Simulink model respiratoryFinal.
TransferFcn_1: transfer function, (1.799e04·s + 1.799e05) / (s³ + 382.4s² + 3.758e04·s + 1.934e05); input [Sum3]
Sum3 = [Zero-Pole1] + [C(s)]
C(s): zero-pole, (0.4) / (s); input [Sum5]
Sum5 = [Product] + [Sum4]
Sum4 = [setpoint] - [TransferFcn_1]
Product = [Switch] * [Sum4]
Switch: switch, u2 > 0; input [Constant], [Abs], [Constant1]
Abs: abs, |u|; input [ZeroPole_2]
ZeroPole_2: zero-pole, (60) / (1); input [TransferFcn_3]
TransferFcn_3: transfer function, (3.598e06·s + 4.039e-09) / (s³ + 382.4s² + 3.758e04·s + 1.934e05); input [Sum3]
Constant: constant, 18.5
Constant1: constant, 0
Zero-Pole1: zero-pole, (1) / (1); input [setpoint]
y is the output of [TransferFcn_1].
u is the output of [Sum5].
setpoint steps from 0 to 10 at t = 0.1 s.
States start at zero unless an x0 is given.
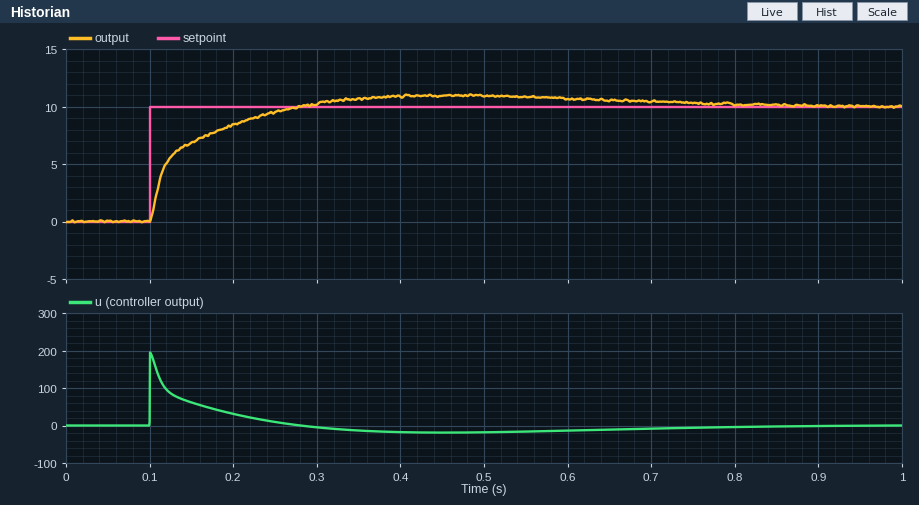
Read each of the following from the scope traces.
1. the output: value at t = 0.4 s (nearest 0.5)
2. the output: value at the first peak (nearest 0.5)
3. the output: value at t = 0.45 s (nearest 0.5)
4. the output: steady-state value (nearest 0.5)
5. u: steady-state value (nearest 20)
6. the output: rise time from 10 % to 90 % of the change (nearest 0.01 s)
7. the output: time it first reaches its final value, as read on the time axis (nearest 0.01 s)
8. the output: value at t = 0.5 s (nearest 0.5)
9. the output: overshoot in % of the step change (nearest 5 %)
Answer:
11.0
11.0
11.0
10.0
0
0.12 s
0.28 s
11.0
10 %
